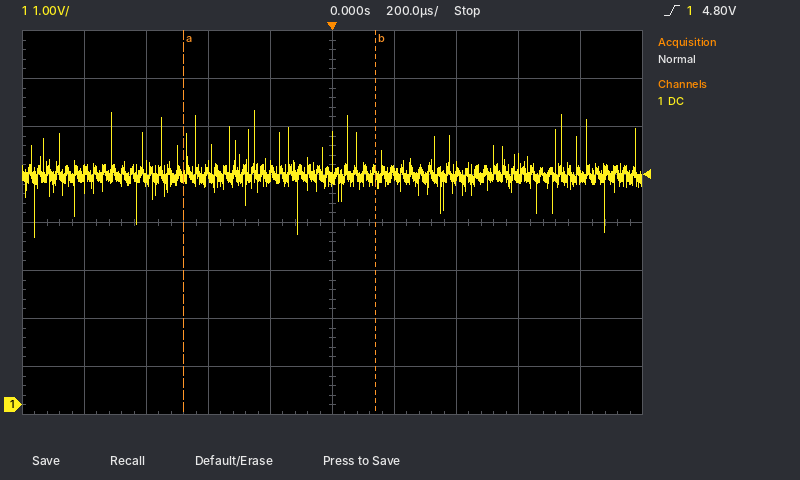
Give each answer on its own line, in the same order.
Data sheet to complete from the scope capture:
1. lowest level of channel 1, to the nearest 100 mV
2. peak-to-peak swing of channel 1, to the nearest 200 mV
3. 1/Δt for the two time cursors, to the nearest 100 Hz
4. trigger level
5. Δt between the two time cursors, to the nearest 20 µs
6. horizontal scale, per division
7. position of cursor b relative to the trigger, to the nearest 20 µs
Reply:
3.5 V
2.6 V
1.6 kHz
4.80 V
620 µs
200 µs
+140 µs
